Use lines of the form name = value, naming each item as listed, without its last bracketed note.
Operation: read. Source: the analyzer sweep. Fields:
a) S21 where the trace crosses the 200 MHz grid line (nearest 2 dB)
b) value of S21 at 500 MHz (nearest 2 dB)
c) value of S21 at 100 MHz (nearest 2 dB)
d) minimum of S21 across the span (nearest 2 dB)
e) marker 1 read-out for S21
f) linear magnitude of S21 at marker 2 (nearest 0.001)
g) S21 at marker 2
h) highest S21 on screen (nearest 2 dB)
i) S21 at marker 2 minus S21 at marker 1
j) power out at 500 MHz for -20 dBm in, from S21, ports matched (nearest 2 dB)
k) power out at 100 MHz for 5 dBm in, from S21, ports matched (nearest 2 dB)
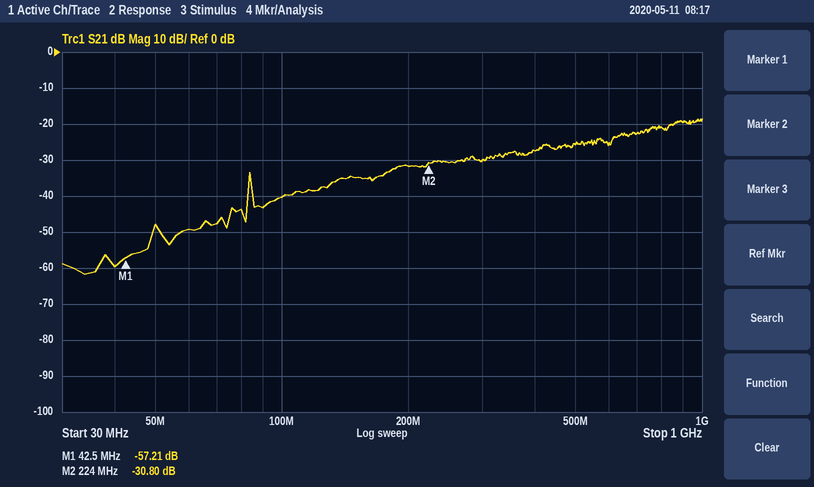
S21 where the trace crosses the 200 MHz grid line = -32 dB
value of S21 at 500 MHz = -26 dB
value of S21 at 100 MHz = -40 dB
minimum of S21 across the span = -62 dB
marker 1 read-out for S21 = -57.21 dB
linear magnitude of S21 at marker 2 = 0.029
S21 at marker 2 = -30.80 dB
highest S21 on screen = -18 dB
S21 at marker 2 minus S21 at marker 1 = 26.41 dB
power out at 500 MHz for -20 dBm in, from S21, ports matched = -46 dBm
power out at 100 MHz for 5 dBm in, from S21, ports matched = -36 dBm
